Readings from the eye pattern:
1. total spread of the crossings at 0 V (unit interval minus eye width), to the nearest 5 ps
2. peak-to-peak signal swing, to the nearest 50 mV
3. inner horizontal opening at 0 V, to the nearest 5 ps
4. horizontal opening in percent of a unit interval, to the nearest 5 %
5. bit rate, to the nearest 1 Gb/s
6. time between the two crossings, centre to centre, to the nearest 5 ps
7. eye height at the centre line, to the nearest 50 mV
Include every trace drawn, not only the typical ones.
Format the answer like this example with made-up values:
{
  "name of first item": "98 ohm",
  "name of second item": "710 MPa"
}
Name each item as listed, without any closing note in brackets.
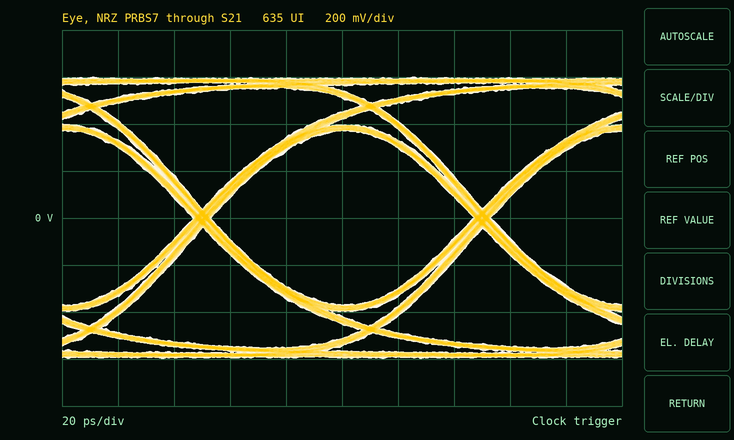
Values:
{
  "total spread of the crossings at 0 V (unit interval minus eye width), to the nearest 5 ps": "5 ps",
  "peak-to-peak signal swing, to the nearest 50 mV": "1.20 V",
  "inner horizontal opening at 0 V, to the nearest 5 ps": "95 ps",
  "horizontal opening in percent of a unit interval, to the nearest 5 %": "95 %",
  "bit rate, to the nearest 1 Gb/s": "10 Gb/s",
  "time between the two crossings, centre to centre, to the nearest 5 ps": "100 ps",
  "eye height at the centre line, to the nearest 50 mV": "750 mV"
}
